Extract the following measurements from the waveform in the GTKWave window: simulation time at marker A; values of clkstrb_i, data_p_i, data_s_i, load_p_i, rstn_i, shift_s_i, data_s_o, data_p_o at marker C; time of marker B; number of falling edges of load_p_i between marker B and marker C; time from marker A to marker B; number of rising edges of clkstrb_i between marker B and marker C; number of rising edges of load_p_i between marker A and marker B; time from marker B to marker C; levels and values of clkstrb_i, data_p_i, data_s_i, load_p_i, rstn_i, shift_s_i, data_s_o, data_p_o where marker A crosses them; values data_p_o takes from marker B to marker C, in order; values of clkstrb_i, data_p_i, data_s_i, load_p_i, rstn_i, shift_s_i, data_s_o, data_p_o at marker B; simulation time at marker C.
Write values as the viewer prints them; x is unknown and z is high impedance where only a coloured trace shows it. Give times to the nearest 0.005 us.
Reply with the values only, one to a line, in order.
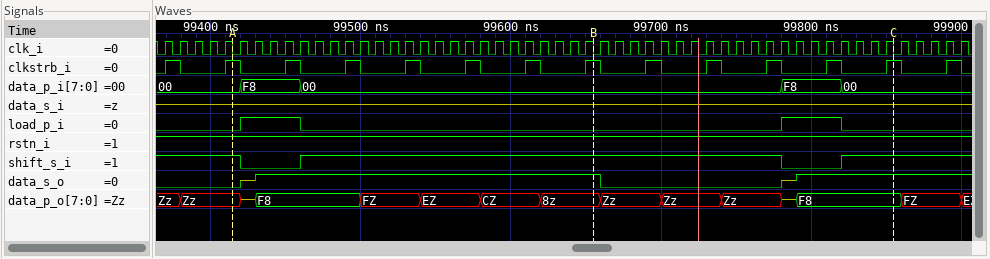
99.415 us
clkstrb_i=1, data_p_i=00, data_s_i=z, load_p_i=0, rstn_i=1, shift_s_i=1, data_s_o=1, data_p_o=F8
99.655 us
1
0.24 us
5
1
0.2 us
clkstrb_i=1, data_p_i=00, data_s_i=z, load_p_i=0, rstn_i=1, shift_s_i=1, data_s_o=0, data_p_o=Zz
8z, Zz, Zz, Zz, z, F8
clkstrb_i=1, data_p_i=00, data_s_i=z, load_p_i=0, rstn_i=1, shift_s_i=1, data_s_o=1, data_p_o=8z
99.855 us
